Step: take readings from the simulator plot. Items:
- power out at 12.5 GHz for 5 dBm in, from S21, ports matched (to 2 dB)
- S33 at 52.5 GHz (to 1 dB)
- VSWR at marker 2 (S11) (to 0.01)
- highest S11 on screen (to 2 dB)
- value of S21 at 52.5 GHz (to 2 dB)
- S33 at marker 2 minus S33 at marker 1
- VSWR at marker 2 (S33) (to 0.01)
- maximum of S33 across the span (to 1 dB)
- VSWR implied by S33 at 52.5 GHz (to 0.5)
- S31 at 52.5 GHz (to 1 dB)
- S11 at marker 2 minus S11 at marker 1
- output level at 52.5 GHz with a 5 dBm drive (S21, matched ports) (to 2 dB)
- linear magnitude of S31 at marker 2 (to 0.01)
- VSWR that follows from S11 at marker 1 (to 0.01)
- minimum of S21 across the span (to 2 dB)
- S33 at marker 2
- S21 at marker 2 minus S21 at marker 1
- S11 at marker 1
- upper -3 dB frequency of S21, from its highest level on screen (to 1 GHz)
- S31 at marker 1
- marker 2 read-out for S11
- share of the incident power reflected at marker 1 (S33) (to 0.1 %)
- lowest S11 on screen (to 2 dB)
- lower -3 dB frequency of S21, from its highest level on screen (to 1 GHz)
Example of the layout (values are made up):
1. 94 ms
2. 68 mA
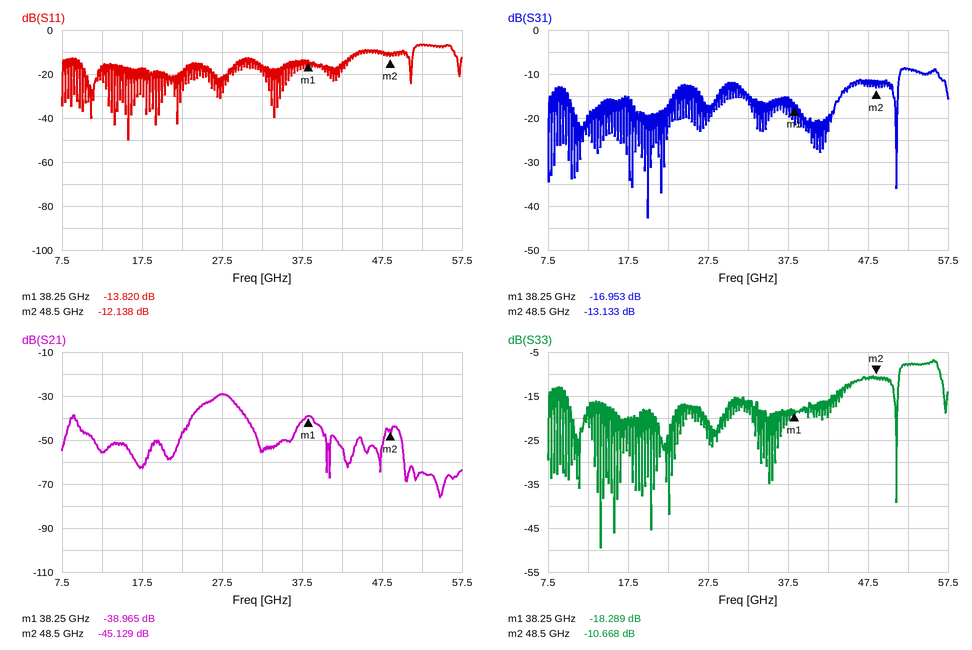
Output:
1. -50 dBm
2. -8 dB
3. 1.66
4. -6 dB
5. -64 dB
6. 7.621 dB
7. 1.83
8. -7 dB
9. 2.5
10. -9 dB
11. 1.682 dB
12. -60 dBm
13. 0.22
14. 1.51
15. -76 dB
16. -10.668 dB
17. -6.164 dB
18. -13.820 dB
19. 29 GHz
20. -16.953 dB
21. -12.138 dB
22. 1.5 %
23. -50 dB
24. 26 GHz
